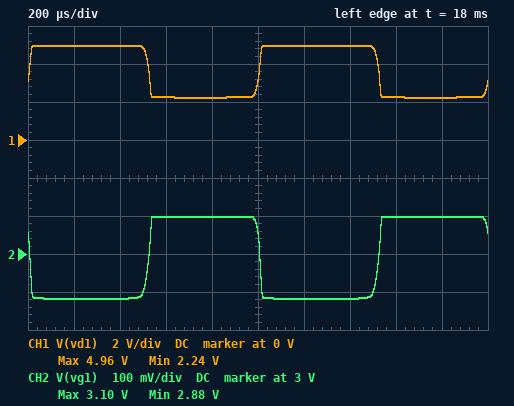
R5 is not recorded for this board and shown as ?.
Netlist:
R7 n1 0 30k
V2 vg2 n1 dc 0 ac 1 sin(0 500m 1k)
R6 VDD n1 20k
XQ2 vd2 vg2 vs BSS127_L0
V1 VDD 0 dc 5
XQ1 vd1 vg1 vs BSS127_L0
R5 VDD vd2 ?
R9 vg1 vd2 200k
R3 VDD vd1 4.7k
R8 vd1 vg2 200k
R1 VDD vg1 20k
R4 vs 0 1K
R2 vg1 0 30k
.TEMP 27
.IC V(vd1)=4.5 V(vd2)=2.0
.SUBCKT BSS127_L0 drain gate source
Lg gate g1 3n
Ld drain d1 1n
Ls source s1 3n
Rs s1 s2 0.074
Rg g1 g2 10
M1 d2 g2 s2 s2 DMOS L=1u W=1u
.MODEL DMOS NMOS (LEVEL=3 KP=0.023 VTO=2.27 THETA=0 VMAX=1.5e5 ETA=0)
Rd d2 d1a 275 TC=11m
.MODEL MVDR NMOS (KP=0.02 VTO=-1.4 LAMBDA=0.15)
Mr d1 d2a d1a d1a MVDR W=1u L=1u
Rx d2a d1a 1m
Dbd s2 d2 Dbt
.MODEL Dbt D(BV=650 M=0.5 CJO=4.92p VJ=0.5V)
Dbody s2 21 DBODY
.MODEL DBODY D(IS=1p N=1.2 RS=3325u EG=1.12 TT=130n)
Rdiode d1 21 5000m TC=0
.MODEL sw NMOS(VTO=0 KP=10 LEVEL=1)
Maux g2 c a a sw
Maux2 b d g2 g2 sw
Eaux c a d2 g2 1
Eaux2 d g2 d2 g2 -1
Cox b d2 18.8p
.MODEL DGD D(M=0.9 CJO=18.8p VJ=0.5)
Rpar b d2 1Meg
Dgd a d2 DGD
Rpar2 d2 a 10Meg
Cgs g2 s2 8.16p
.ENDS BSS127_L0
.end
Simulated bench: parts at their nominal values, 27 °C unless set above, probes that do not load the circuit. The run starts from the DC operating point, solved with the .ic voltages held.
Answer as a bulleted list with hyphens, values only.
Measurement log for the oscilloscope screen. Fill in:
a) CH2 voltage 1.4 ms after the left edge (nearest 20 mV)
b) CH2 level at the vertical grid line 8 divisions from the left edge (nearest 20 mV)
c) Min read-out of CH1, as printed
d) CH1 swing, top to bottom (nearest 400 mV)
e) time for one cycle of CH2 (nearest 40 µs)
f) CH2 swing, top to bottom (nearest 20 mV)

- 2.88 V
- 3.10 V
- 2.24 V
- 2.8 V
- 1.00 ms
- 220 mV
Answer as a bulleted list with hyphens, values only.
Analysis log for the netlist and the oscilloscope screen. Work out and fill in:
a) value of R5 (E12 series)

- 6.8 kΩ
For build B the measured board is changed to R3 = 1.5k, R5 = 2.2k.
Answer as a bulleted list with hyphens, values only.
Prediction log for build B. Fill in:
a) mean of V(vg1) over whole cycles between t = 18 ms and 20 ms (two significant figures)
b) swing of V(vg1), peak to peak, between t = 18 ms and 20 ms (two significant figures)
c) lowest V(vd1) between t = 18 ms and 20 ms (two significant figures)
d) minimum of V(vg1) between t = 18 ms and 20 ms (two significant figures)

- 3.1 V
- 120 mV
- 4.1 V
- 3.0 V
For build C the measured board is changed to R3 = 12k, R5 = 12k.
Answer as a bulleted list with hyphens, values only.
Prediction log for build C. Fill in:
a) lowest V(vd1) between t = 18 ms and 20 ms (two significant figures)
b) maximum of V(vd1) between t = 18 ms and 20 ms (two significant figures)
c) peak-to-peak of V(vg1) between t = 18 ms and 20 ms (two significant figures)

- 540 mV
- 3.6 V
- 210 mV
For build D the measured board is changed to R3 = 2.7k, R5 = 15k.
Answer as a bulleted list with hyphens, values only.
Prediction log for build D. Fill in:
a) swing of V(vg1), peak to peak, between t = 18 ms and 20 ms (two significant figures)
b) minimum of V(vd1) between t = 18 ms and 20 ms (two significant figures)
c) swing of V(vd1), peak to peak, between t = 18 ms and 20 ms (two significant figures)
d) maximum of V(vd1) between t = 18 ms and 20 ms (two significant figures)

- 240 mV
- 3.4 V
- 1.2 V
- 4.5 V
